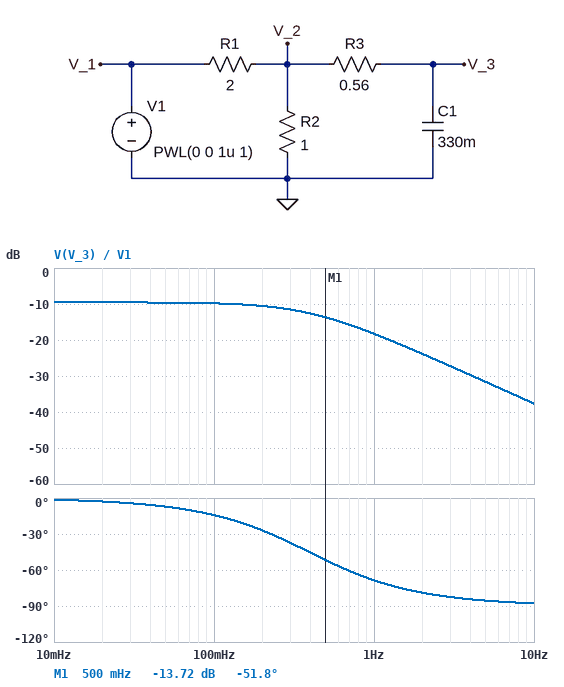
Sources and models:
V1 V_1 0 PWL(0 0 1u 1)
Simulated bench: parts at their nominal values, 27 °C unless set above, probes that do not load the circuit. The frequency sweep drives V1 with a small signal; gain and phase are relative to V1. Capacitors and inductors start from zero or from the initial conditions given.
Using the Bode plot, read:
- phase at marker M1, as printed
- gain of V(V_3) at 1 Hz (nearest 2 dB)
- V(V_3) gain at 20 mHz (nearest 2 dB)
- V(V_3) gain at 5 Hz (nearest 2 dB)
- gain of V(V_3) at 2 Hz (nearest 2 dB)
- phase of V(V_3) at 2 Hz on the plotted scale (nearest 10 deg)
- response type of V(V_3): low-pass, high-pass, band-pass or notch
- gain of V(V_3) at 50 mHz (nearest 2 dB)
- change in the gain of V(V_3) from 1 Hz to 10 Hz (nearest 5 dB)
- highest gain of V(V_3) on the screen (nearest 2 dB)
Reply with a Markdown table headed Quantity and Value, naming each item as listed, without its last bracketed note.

| Quantity | Value |
|---|---|
| phase at marker M1, as printed | -51.8 deg |
| gain of V(V_3) at 1 Hz | -18 dB |
| V(V_3) gain at 20 mHz | -10 dB |
| V(V_3) gain at 5 Hz | -32 dB |
| gain of V(V_3) at 2 Hz | -24 dB |
| phase of V(V_3) at 2 Hz on the plotted scale | -80 deg |
| response type of V(V_3): low-pass, high-pass, band-pass or notch | low-pass |
| gain of V(V_3) at 50 mHz | -10 dB |
| change in the gain of V(V_3) from 1 Hz to 10 Hz | -20 dB |
| highest gain of V(V_3) on the screen | -10 dB |
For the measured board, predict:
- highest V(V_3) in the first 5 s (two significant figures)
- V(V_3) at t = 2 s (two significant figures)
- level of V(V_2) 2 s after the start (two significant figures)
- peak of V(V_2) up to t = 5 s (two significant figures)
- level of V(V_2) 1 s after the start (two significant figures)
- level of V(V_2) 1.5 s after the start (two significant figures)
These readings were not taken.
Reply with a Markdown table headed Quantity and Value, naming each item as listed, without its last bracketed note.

| Quantity | Value |
|---|---|
| highest V(V_3) in the first 5 s | 330 mV |
| V(V_3) at t = 2 s | 330 mV |
| level of V(V_2) 2 s after the start | 330 mV |
| peak of V(V_2) up to t = 5 s | 330 mV |
| level of V(V_2) 1 s after the start | 320 mV |
| level of V(V_2) 1.5 s after the start | 330 mV |
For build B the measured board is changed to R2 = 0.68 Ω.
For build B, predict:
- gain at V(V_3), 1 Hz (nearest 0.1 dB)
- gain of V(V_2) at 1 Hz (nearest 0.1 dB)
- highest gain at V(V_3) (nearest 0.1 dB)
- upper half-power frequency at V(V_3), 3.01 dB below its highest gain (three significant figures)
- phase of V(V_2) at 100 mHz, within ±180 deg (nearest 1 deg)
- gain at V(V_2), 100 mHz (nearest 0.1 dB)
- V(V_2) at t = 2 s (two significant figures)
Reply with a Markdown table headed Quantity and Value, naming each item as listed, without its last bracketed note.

| Quantity | Value |
|---|---|
| gain at V(V_3), 1 Hz | -19.6 dB |
| gain of V(V_2) at 1 Hz | -15.9 dB |
| highest gain at V(V_3) | -11.9 dB |
| upper half-power frequency at V(V_3), 3.01 dB below its highest gain | 452 mHz |
| phase of V(V_2) at 100 mHz, within ±180 deg | -6 deg |
| gain at V(V_2), 100 mHz | -12.1 dB |
| V(V_2) at t = 2 s | 250 mV |
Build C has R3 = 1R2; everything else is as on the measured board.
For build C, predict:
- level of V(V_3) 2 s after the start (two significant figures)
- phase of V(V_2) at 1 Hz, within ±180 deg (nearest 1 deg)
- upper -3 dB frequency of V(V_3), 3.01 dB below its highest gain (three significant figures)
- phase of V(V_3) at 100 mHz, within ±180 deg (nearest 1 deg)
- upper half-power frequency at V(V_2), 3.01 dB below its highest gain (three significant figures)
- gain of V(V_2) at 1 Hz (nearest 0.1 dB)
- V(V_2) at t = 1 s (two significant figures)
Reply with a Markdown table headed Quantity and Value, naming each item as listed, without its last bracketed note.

| Quantity | Value |
|---|---|
| level of V(V_3) 2 s after the start | 320 mV |
| phase of V(V_2) at 1 Hz, within ±180 deg | -7 deg |
| upper -3 dB frequency of V(V_3), 3.01 dB below its highest gain | 258 mHz |
| phase of V(V_3) at 100 mHz, within ±180 deg | -21 deg |
| upper half-power frequency at V(V_2), 3.01 dB below its highest gain | 620 mHz |
| gain of V(V_2) at 1 Hz | -13.0 dB |
| V(V_2) at t = 1 s | 310 mV |
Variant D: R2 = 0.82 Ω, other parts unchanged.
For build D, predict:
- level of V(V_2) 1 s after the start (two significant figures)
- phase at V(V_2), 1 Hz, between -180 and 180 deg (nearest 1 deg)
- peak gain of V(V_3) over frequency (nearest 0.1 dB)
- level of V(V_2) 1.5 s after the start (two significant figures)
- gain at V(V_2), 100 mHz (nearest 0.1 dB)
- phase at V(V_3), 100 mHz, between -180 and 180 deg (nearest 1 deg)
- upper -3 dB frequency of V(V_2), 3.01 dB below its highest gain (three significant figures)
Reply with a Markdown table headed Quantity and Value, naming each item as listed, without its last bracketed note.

| Quantity | Value |
|---|---|
| level of V(V_2) 1 s after the start | 280 mV |
| phase at V(V_2), 1 Hz, between -180 and 180 deg | -18 deg |
| peak gain of V(V_3) over frequency | -10.7 dB |
| level of V(V_2) 1.5 s after the start | 290 mV |
| gain at V(V_2), 100 mHz | -10.9 dB |
| phase at V(V_3), 100 mHz, between -180 and 180 deg | -13 deg |
| upper -3 dB frequency of V(V_2), 3.01 dB below its highest gain | 587 mHz |
